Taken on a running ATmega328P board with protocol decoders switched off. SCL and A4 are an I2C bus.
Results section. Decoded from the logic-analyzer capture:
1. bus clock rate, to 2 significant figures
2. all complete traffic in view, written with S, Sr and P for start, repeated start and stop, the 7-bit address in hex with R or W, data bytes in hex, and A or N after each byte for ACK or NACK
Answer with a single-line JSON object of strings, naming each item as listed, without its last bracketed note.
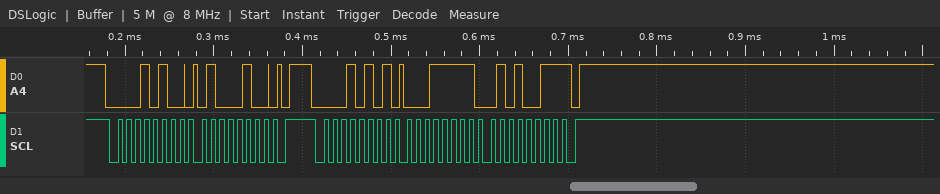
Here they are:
{"bus clock rate, to 2 significant figures": "100 kHz", "all complete traffic in view, written with S, Sr and P for start, repeated start and stop, the 7-bit address in hex with R or W, data bytes in hex, and A or N after each byte for ACK or NACK": "S 0AW A 44 A P S 0AR A 1F A 53 N P"}
